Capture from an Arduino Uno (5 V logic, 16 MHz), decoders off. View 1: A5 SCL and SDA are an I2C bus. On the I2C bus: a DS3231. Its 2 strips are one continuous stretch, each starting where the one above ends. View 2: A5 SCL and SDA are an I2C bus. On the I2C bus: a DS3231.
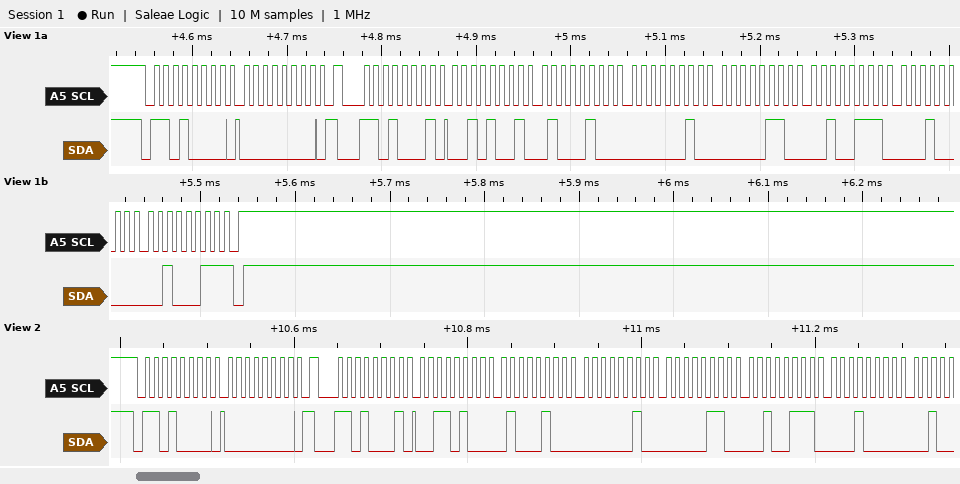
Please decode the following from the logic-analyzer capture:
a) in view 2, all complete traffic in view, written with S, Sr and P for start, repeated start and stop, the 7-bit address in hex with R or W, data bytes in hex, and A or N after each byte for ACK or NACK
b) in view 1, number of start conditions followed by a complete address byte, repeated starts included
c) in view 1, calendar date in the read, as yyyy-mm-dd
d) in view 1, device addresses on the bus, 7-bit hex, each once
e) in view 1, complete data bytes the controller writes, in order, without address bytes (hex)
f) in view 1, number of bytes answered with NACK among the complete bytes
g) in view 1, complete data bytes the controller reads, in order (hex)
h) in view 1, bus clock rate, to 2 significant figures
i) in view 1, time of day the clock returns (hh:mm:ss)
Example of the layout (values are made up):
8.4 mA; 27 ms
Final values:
S 68W A 00 A Sr 68R A 34 A 44 A 02 A 06 A 27 A 10 A; 2; 2023-10-27; 0x68; 00; 1; 29 44 02 06 27 10 23; 100 kHz; 02:44:29
